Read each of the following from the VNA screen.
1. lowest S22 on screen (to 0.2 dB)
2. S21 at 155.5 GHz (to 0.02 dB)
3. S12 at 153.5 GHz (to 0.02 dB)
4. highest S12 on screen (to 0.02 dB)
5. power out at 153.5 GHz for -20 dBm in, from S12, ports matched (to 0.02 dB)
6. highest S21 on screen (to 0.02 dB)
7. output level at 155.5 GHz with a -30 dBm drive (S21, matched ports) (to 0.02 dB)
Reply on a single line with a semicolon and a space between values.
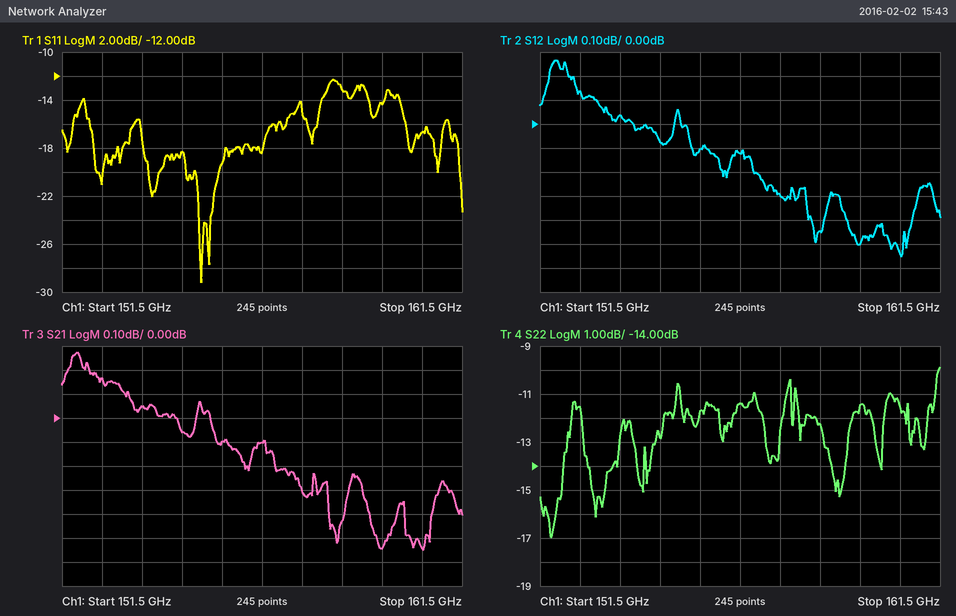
-17.0 dB; -0.10 dB; 0.04 dB; 0.26 dB; -19.96 dBm; 0.28 dB; -30.10 dBm
